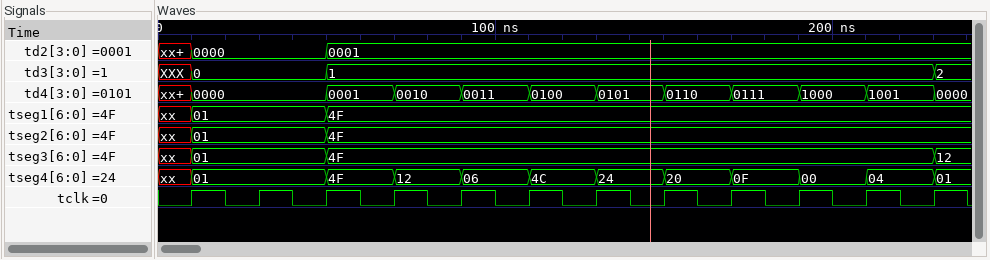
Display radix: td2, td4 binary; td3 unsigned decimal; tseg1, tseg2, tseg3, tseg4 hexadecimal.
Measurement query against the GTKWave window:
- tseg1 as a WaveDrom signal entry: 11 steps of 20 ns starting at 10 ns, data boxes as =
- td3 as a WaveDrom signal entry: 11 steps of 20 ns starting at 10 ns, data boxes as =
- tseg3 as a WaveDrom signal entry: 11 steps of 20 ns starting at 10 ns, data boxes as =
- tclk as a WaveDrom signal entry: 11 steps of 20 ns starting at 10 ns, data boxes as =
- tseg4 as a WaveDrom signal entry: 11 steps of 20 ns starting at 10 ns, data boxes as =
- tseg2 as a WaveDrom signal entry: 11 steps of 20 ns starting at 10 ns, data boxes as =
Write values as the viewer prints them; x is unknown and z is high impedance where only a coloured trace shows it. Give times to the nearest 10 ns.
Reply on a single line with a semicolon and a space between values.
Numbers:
{name: 'tseg1', wave: '=.=........', data: '01 4F'}; {name: 'td3', wave: '=.=........', data: '0 1'}; {name: 'tseg3', wave: '=.=........', data: '01 4F'}; {name: 'tclk', wave: 'p..........'}; {name: 'tseg4', wave: '=.=========', data: '01 4F 12 06 4C 24 20 0F 00 04'}; {name: 'tseg2', wave: '=.=........', data: '01 4F'}
